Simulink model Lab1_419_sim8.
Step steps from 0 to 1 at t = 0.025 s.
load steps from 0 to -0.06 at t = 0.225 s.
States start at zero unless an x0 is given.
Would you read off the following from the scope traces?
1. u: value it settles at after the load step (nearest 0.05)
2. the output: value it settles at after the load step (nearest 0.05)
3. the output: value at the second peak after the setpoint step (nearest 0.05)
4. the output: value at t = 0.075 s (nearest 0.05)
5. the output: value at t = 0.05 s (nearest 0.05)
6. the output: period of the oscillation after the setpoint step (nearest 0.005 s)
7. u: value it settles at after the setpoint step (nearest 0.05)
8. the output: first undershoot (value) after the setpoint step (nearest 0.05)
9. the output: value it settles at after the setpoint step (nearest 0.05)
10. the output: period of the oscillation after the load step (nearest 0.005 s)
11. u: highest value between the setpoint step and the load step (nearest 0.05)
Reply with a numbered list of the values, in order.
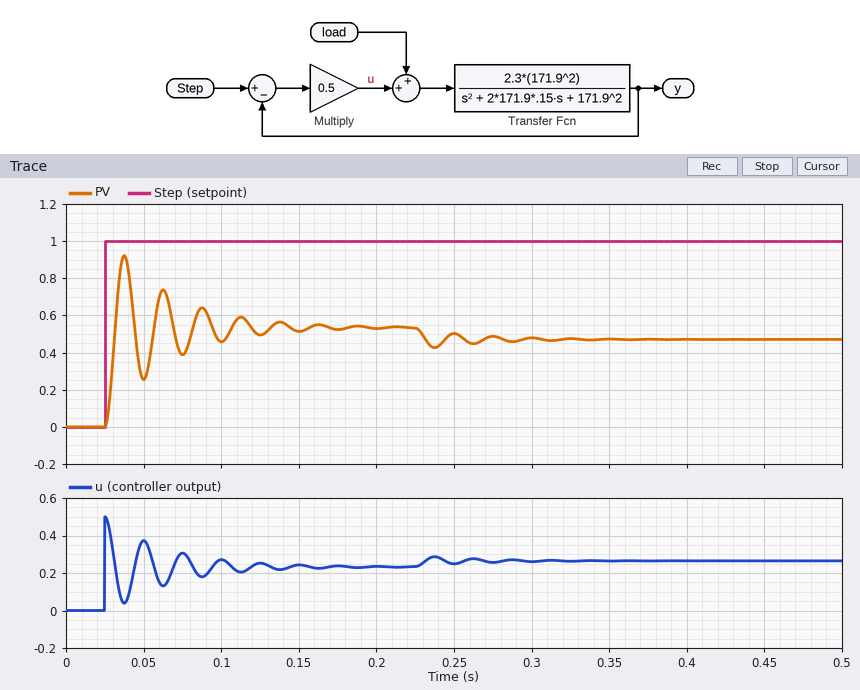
1. 0.25
2. 0.45
3. 0.75
4. 0.40
5. 0.25
6. 0.025 s
7. 0.25
8. 0.25
9. 0.55
10. 0.025 s
11. 0.50
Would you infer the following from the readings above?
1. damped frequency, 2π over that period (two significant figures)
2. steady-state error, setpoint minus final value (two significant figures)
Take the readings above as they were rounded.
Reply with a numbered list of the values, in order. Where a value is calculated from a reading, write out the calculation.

1. 2π / 0.025 = 250 rad/s
2. 1 - 0.55 = 0.45
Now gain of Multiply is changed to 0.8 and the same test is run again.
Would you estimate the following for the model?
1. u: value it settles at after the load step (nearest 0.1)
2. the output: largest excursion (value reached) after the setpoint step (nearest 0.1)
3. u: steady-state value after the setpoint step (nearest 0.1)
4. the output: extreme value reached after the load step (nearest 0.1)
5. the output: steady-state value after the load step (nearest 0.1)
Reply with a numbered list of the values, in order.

1. 0.3
2. 1.1
3. 0.3
4. 0.6
5. 0.6
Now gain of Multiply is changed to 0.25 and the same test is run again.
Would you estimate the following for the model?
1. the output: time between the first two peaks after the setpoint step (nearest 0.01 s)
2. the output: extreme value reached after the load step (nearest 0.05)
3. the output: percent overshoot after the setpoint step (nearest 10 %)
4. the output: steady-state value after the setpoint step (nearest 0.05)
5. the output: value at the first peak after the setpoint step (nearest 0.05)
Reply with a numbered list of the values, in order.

1. 0.03 s
2. 0.20
3. 70 %
4. 0.35
5. 0.60
